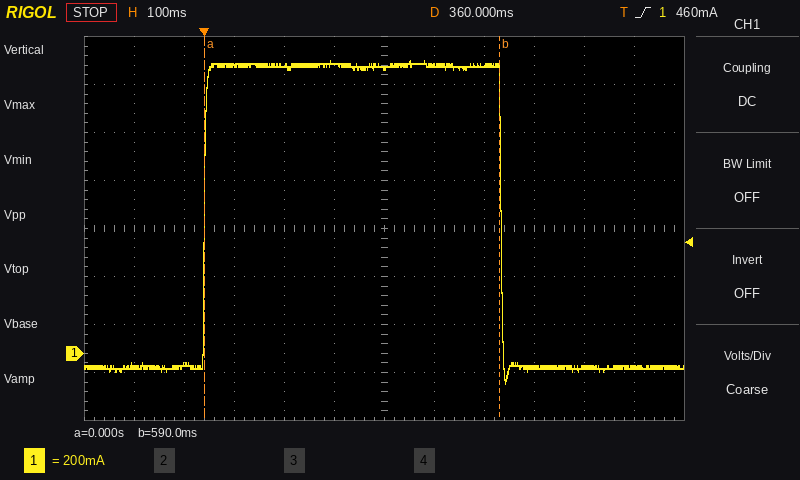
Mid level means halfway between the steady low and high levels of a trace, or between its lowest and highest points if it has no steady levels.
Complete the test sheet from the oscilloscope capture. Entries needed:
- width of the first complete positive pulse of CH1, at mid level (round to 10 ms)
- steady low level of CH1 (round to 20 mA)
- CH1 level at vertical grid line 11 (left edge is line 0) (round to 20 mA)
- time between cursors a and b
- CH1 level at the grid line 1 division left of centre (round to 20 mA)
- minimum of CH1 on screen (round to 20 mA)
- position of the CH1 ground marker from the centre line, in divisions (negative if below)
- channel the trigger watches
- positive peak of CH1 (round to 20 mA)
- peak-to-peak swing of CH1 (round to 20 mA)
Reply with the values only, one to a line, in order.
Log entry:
590 ms
-60 mA
-60 mA
590 ms
1.20 A
-120 mA
-2.6 div
CH1
1.22 A
1.34 A
